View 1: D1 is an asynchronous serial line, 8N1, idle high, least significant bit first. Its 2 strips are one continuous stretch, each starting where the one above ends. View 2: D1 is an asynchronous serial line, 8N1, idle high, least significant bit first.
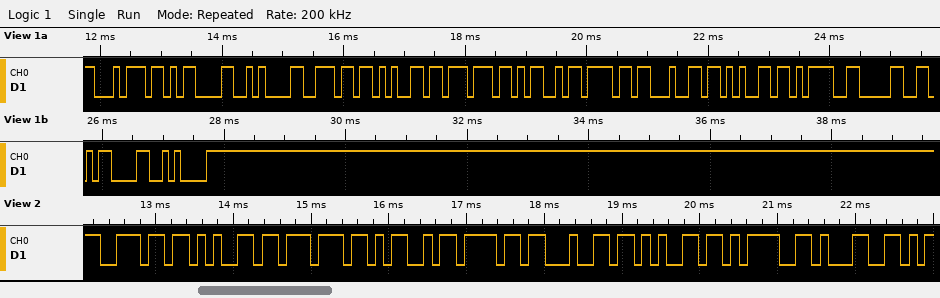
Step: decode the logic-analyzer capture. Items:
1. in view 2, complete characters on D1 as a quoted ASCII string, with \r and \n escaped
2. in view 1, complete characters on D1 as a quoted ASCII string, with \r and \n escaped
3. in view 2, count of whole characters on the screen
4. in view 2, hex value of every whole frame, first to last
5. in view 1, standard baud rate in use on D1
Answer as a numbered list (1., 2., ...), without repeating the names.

1. "newMode=1"
2. "t\r\nnewMode=0\r\n"
3. 9
4. 6E 65 77 4D 6F 64 65 3D 31
5. 9600 baud
